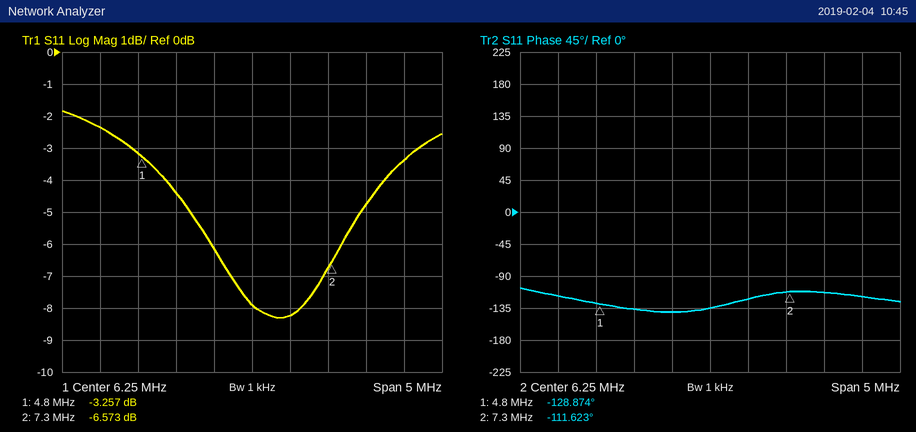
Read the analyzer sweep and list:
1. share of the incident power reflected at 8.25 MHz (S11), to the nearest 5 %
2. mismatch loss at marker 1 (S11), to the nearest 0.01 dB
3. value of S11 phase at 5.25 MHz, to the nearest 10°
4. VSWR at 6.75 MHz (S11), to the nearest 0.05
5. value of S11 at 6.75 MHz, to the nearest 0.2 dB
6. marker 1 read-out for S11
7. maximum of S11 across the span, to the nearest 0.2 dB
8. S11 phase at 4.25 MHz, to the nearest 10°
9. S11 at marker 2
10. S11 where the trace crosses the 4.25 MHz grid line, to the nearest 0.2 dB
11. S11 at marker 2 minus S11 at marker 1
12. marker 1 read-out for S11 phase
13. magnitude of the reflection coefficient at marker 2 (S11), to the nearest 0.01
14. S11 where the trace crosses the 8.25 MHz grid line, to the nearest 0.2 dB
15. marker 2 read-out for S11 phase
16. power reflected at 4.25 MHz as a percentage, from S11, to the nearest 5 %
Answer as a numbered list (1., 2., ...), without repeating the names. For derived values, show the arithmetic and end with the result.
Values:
1. 10^(-3.4/10) ≈ 45.7 %, so 45 % to the nearest 5 %
2. −10 log10(1 − 10^(-3.257/10)) ≈ 2.78 dB
3. -140°
4. |Γ| = 10^(-8.2/20) = 0.3890; VSWR = (1 + 0.3890)/(1 − 0.3890) ≈ 2.27, so 2.25 to the nearest 0.05
5. -8.2 dB
6. -3.257 dB
7. -1.8 dB
8. -120°
9. -6.573 dB
10. -2.4 dB
11. -6.573 − (-3.257) = -3.316 dB
12. -128.874°
13. 10^(-6.573/20) ≈ 0.47
14. -3.4 dB
15. -111.623°
16. 10^(-2.4/10) ≈ 57.5 %, so 60 % to the nearest 5 %
